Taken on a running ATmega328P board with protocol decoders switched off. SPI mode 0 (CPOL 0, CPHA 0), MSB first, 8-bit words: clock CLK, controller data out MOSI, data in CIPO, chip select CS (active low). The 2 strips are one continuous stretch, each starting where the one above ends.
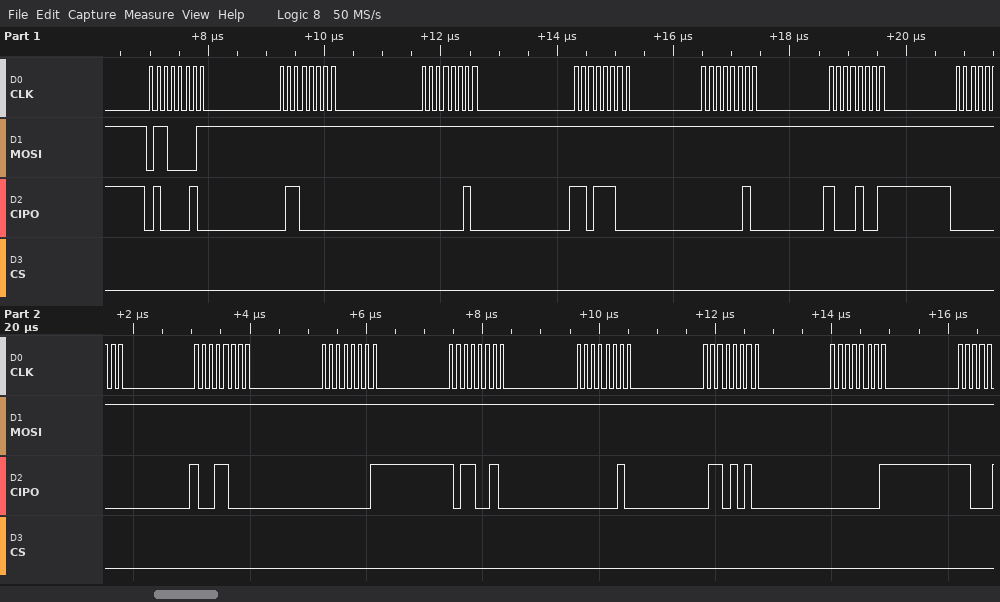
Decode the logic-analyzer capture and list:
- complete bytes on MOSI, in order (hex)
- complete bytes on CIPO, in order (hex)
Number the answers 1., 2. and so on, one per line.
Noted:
1. 61 FF FF FF FF FF FF FF FF FF FF FF FF
2. 42 60 02 DC 02 89 00 98 01 B2 02 6A 01
